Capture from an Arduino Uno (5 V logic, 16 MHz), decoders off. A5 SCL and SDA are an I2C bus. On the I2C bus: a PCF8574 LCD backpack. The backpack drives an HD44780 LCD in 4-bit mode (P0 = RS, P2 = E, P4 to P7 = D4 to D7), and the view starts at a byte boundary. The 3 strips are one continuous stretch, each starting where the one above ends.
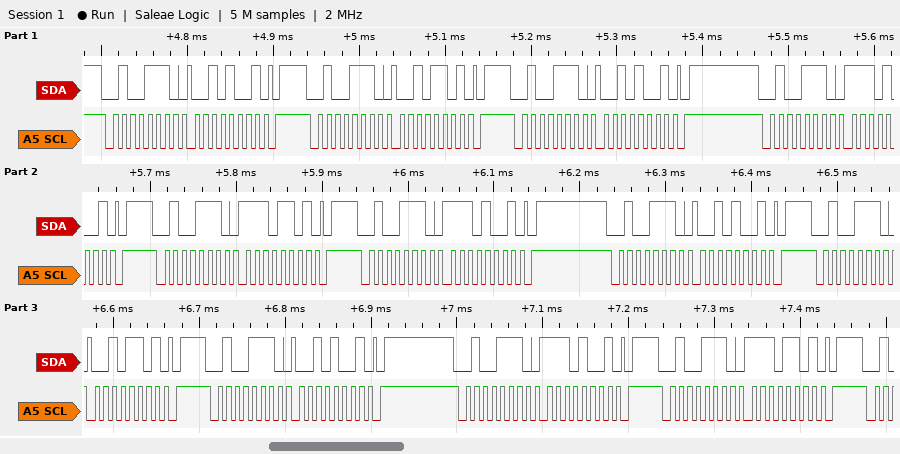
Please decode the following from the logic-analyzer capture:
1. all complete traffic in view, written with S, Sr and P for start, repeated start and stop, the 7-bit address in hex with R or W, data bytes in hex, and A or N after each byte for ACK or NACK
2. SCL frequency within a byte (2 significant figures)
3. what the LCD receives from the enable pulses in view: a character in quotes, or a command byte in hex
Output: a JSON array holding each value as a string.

["S 27W A 29 A P S 27W A 2D A P S 27W A 29 A P S 27W A E9 A P S 27W A ED A P S 27W A E9 A P S 27W A 29 A P S 27W A 2D A P S 27W A 29 A P S 27W A E9 A P S 27W A ED A P", "100 kHz", "'.'"]
